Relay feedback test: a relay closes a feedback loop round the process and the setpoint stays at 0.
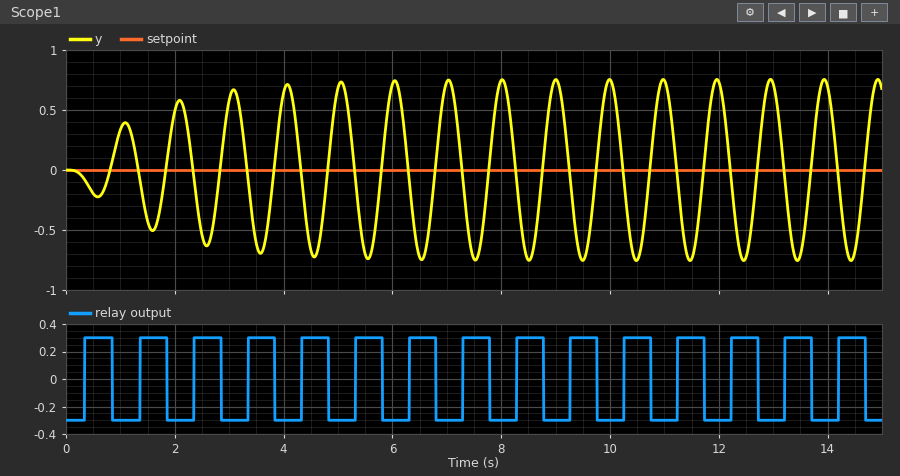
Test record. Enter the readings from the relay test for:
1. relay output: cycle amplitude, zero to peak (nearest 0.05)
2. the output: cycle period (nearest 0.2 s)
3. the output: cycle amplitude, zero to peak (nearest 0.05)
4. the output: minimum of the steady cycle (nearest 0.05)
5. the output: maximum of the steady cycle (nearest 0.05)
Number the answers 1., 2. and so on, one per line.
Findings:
1. 0.30
2. 1.0 s
3. 0.75
4. -0.75
5. 0.75
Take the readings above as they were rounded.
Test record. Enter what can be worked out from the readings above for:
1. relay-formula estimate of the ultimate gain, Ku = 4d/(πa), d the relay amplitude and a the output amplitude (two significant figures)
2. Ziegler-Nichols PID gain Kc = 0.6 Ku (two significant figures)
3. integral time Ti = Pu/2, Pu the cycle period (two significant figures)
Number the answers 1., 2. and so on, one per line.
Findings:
1. 0.51
2. 0.31
3. 0.50 s
